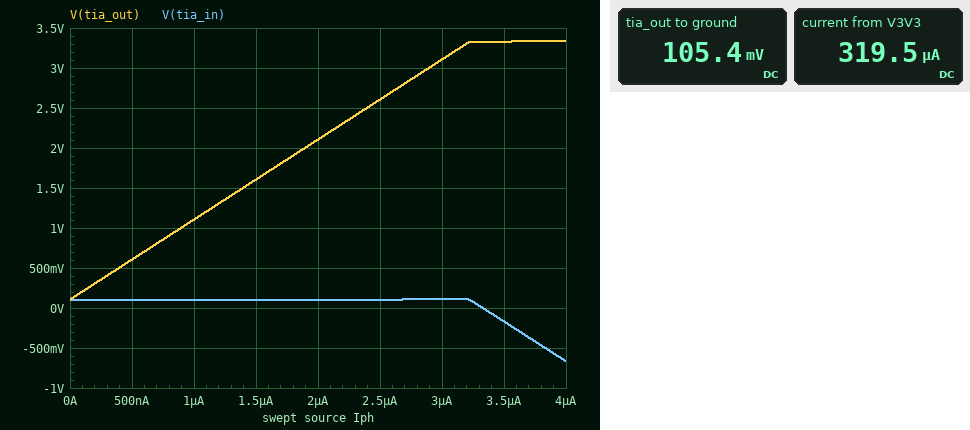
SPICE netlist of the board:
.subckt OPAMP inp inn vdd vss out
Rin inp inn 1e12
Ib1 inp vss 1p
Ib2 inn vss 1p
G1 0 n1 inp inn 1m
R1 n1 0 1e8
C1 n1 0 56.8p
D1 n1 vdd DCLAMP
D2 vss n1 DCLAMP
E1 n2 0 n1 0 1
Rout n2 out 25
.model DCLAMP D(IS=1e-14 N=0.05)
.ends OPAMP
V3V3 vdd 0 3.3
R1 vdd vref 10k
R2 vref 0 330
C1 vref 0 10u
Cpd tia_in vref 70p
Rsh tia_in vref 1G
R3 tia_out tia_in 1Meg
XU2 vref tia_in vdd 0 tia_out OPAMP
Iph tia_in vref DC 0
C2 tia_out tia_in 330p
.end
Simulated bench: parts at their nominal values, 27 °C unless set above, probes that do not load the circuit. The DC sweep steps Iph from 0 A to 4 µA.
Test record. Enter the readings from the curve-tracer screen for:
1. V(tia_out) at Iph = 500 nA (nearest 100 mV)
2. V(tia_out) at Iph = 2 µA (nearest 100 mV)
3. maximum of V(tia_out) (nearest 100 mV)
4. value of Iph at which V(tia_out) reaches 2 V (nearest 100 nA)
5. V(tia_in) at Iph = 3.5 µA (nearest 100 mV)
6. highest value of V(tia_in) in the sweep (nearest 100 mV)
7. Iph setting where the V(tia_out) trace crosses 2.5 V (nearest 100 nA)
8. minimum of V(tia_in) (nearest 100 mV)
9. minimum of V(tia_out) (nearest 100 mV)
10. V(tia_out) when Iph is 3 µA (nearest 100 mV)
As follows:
600 mV
2.1 V
3.3 V
1.9 µA
-200 mV
100 mV
2.4 µA
-700 mV
100 mV
3.1 V
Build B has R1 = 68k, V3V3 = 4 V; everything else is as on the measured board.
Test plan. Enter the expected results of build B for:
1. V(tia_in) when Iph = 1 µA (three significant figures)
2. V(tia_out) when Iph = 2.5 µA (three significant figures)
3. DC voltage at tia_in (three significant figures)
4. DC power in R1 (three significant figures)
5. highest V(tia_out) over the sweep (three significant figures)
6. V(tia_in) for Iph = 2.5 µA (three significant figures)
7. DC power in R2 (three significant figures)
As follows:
19.6 mV
2.52 V
19.3 mV
233 µW
4.02 V
20.1 mV
1.13 µW
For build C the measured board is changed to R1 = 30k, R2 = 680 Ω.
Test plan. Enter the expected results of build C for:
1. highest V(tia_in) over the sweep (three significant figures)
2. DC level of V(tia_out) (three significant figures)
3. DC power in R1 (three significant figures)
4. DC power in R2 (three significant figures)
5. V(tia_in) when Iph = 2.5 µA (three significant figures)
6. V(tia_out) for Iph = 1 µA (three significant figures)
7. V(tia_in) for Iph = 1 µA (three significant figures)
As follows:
75.3 mV
73.1 mV
347 µW
7.87 µW
74.8 mV
1.07 V
73.8 mV
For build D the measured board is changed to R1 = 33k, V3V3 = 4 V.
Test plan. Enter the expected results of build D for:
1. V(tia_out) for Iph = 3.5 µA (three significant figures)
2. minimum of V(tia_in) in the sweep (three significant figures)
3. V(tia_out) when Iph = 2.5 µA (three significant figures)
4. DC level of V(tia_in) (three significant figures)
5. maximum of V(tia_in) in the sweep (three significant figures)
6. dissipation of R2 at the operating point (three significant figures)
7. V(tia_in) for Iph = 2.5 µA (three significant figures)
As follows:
3.54 V
27.1 mV
2.54 V
39.6 mV
40.9 mV
4.75 µW
40.4 mV
